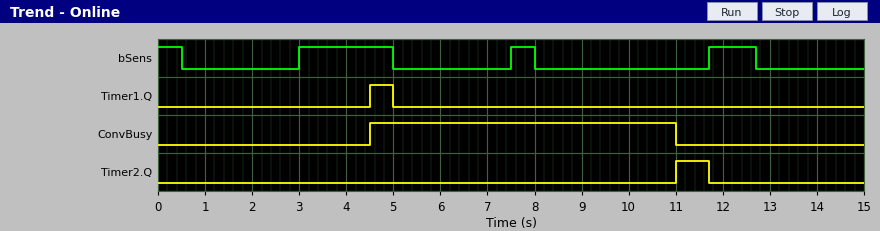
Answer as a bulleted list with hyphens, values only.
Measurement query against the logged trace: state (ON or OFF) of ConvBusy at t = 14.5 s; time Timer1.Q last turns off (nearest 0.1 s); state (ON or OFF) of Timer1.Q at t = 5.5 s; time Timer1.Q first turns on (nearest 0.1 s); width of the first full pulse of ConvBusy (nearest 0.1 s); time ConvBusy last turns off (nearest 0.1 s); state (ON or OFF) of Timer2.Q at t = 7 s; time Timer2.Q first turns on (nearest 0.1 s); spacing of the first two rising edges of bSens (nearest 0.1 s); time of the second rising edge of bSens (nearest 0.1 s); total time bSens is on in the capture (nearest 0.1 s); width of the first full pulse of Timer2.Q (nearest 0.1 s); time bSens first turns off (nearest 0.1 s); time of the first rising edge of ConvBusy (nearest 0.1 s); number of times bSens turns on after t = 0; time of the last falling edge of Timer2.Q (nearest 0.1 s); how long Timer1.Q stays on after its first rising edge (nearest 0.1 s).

- OFF
- 5.0 s
- OFF
- 4.5 s
- 6.5 s
- 11.0 s
- OFF
- 11.0 s
- 4.5 s
- 7.5 s
- 4.0 s
- 0.7 s
- 0.5 s
- 4.5 s
- 3
- 11.7 s
- 0.5 s
